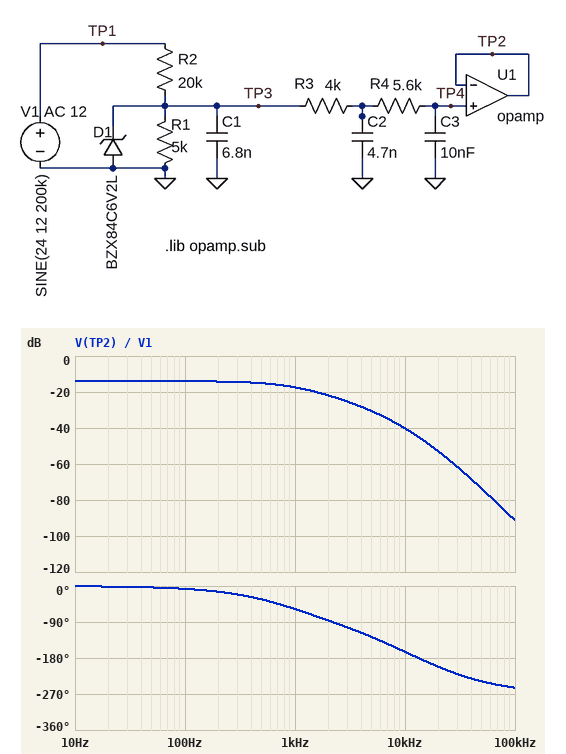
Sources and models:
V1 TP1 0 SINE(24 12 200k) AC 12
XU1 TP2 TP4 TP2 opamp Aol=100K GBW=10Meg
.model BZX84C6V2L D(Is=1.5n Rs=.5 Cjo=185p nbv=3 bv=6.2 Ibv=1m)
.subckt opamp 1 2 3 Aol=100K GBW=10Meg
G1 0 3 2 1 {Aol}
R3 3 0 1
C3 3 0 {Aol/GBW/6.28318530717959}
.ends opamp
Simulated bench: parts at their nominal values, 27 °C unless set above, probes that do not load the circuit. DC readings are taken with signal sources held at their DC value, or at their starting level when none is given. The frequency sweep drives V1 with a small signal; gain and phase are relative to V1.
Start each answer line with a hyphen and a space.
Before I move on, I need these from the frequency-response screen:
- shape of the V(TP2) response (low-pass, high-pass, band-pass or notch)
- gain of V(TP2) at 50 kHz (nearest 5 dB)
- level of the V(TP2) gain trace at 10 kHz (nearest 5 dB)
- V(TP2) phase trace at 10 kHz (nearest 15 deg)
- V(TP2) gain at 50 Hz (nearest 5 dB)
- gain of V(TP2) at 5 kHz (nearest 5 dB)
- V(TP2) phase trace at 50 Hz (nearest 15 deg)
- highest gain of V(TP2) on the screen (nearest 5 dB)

- low-pass
- -75 dB
- -40 dB
- -165 deg
- -15 dB
- -30 dB
- 0 deg
- -15 dB
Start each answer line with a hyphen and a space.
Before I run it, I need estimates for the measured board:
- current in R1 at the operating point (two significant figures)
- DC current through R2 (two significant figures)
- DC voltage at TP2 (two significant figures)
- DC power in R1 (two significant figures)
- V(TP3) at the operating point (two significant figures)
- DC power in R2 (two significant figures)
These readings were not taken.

- 960 µA
- 960 µA
- 4.8 V
- 4.6 mW
- 4.8 V
- 18 mW
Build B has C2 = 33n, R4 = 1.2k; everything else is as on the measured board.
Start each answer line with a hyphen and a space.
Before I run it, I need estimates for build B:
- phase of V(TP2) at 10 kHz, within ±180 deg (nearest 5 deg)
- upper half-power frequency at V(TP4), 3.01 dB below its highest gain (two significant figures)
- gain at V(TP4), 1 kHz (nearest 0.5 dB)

- -155 deg
- 440 Hz
- -22.0 dB
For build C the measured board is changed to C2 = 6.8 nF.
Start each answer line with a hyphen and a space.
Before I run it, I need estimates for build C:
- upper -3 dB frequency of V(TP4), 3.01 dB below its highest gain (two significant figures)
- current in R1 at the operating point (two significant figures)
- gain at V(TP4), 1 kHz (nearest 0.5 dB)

- 850 Hz
- 960 µA
- -18.0 dB
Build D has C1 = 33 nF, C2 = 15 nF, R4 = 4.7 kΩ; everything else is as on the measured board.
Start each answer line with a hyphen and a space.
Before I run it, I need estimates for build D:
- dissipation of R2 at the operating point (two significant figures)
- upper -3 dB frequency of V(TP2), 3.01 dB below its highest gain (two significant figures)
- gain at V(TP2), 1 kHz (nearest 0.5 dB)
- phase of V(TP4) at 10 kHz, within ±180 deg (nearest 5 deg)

- 18 mW
- 510 Hz
- -21.0 dB
- 145 deg
